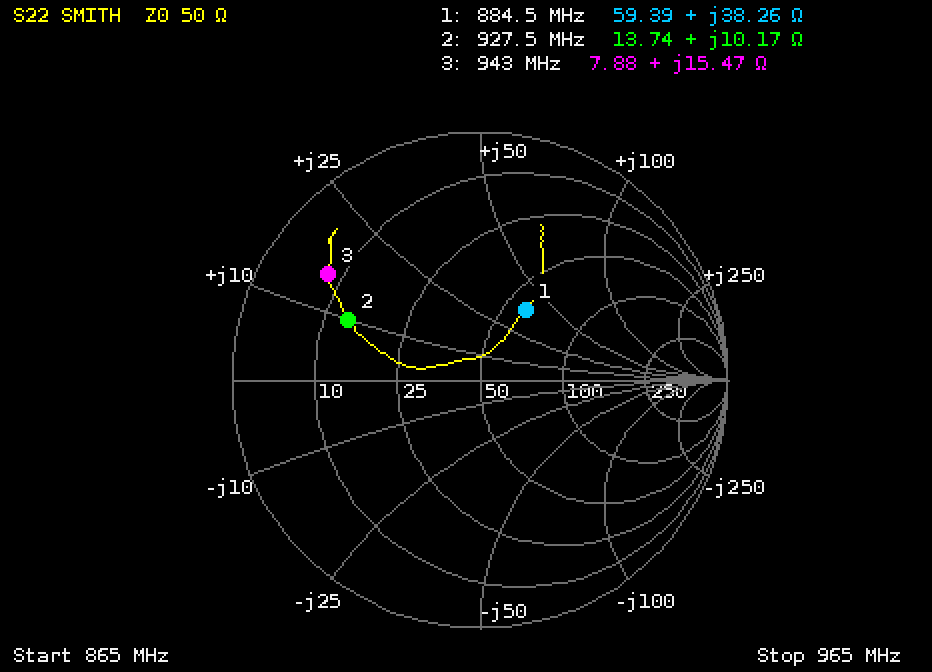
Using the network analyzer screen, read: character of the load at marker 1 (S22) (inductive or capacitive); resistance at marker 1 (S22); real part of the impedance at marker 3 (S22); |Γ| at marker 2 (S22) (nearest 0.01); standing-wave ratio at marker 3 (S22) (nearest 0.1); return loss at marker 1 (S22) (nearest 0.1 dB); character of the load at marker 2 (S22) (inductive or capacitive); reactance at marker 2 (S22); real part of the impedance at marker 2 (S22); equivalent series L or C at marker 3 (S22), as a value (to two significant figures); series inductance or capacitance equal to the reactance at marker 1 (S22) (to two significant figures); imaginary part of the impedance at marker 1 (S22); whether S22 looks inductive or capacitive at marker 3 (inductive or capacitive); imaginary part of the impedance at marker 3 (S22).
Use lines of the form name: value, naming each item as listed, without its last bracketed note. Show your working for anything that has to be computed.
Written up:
character of the load at marker 1 (S22): inductive
resistance at marker 1: 59.39 Ω
real part of the impedance at marker 3: 7.88 Ω
|Γ| at marker 2 (S22): 0.58
standing-wave ratio at marker 3 (S22): 7.0
return loss at marker 1 (S22): 9.4 dB
character of the load at marker 2 (S22): inductive
reactance at marker 2: +10.17 Ω
real part of the impedance at marker 2: 13.74 Ω
equivalent series L or C at marker 3 (S22), as a value: L = 15.47 Ω/(2π × 943 MHz) ≈ 2.6 nH
series inductance or capacitance equal to the reactance at marker 1 (S22): L = 38.26 Ω/(2π × 884.5 MHz) ≈ 6.9 nH
imaginary part of the impedance at marker 1: +38.26 Ω
whether S22 looks inductive or capacitive at marker 3: inductive
imaginary part of the impedance at marker 3: +15.47 Ω
